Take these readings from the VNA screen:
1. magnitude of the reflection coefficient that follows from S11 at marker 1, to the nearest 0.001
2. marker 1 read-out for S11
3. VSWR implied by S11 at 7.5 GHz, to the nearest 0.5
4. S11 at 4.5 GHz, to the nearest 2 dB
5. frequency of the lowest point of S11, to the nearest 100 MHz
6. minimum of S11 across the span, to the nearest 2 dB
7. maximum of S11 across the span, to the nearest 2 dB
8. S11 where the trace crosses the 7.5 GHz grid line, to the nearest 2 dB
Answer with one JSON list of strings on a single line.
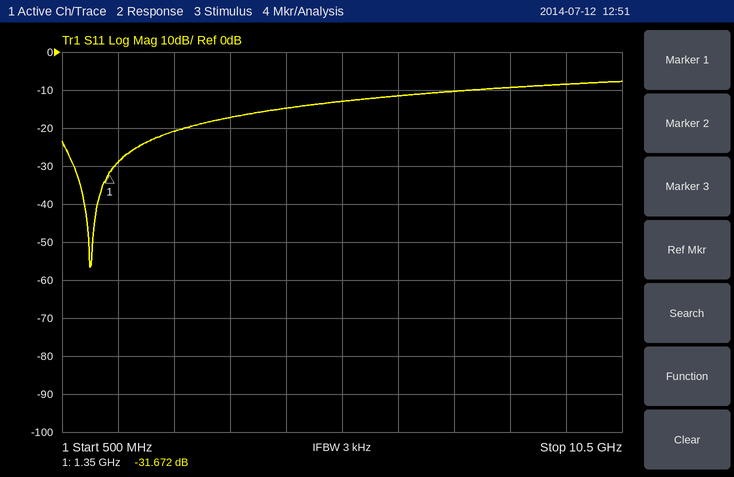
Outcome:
["0.026", "-31.672 dB", "2.0", "-14 dB", "1.0 GHz", "-56 dB", "-8 dB", "-10 dB"]
